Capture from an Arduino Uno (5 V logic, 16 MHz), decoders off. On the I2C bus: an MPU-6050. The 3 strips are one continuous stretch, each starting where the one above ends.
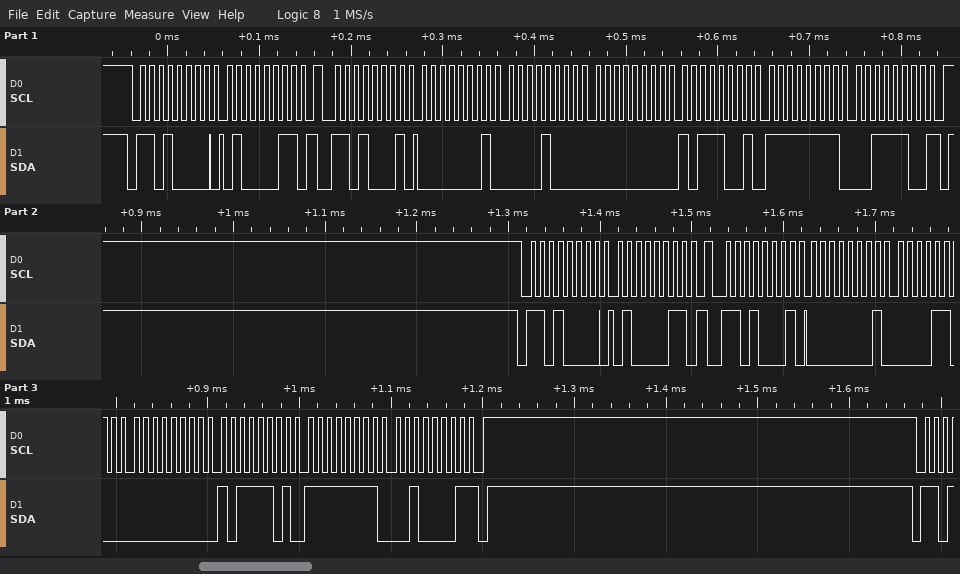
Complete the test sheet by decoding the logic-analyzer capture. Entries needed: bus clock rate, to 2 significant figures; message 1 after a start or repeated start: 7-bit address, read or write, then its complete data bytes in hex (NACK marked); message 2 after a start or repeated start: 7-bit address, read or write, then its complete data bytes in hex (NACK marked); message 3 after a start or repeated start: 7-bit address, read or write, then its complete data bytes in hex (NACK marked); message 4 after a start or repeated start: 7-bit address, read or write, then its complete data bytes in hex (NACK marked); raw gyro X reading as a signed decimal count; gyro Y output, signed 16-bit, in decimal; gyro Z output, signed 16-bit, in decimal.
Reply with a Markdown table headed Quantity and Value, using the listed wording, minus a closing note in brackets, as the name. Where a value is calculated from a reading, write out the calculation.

| Quantity | Value |
|---|---|
| bus clock rate, to 2 significant figures | 100 kHz |
| message 1 after a start or repeated start: 7-bit address, read or write, then its complete data bytes in hex | 0x68 write: 43 |
| message 2 after a start or repeated start: 7-bit address, read or write, then its complete data bytes in hex | 0x68 read: 01 08 00 B9 FF 3C NACK |
| message 3 after a start or repeated start: 7-bit address, read or write, then its complete data bytes in hex | 0x68 write: 43 |
| message 4 after a start or repeated start: 7-bit address, read or write, then its complete data bytes in hex | 0x68 read: 01 0C 00 BD FF 21 NACK |
| raw gyro X reading as a signed decimal count | 0x0108 = 264 |
| gyro Y output, signed 16-bit, in decimal | 0x00B9 = 185 |
| gyro Z output, signed 16-bit, in decimal | 0xFF3C = -196 |
